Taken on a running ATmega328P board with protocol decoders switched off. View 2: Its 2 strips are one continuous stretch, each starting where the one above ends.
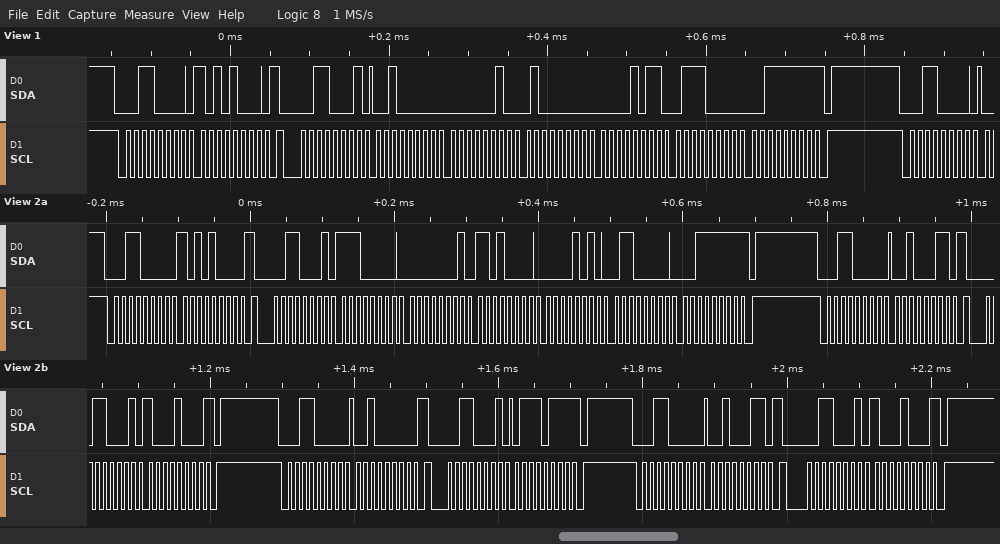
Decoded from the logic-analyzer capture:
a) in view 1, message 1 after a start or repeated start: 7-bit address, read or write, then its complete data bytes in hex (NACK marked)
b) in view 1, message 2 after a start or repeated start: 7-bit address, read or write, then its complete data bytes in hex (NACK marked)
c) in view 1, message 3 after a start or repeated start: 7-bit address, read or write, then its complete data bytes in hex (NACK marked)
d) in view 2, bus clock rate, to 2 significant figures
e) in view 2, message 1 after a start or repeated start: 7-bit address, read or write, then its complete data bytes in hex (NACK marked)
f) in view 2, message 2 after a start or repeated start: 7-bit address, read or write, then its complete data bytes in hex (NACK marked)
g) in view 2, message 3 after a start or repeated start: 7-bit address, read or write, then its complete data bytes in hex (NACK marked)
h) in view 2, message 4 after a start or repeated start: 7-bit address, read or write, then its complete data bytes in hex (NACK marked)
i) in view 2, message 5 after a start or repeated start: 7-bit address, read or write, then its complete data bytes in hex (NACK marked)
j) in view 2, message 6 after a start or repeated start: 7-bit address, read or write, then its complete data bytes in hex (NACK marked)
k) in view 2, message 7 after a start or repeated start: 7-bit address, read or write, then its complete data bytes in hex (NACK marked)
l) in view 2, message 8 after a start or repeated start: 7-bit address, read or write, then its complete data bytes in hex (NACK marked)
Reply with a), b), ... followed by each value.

a) 0x18 write: A8
b) 0x18 read: 20 02 40 0B 70 3F NACK
c) 0x18 write
d) 100 kHz
e) 0x18 write: A8
f) 0x18 read: E0 01 D0 0A 60 3F NACK
g) 0x18 write: 23
h) 0x18 read: 88 NACK
i) 0x18 write: 20
j) 0x18 read: 77 NACK
k) 0x18 write: 23
l) 0x18 read: 88 NACK
